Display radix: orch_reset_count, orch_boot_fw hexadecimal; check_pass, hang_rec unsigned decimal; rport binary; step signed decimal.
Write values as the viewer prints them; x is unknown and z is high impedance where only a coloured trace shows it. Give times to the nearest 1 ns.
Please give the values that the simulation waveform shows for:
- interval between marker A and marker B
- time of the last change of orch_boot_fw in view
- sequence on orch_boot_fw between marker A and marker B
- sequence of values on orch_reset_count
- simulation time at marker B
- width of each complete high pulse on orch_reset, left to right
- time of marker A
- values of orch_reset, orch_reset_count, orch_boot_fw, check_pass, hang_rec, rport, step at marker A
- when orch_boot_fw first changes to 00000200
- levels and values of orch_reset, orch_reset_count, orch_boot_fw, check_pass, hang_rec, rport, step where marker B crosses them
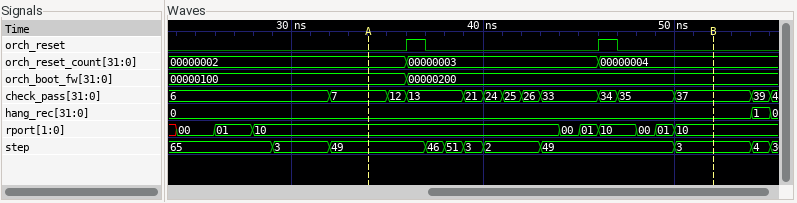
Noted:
18 ns
36 ns
00000100, 00000200
00000002, 00000003, 00000004
52 ns
1 ns, 1 ns
34 ns
orch_reset=0, orch_reset_count=00000002, orch_boot_fw=00000100, check_pass=7, hang_rec=0, rport=10, step=49
36 ns
orch_reset=0, orch_reset_count=00000004, orch_boot_fw=00000200, check_pass=37, hang_rec=0, rport=10, step=3
